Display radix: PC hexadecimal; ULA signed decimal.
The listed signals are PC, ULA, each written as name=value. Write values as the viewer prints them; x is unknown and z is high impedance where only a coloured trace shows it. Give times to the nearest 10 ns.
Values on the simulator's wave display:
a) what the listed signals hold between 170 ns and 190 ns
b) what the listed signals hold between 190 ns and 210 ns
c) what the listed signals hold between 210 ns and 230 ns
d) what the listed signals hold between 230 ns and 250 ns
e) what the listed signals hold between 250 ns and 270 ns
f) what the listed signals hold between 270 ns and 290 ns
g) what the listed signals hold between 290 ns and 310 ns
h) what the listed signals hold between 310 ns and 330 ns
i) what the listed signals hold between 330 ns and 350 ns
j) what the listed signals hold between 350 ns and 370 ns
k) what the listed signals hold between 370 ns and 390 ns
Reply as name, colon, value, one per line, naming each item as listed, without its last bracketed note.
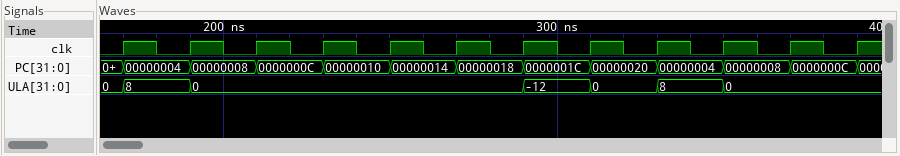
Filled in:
what the listed signals hold between 170 ns and 190 ns: PC=00000004, ULA=8
what the listed signals hold between 190 ns and 210 ns: PC=00000008, ULA=0
what the listed signals hold between 210 ns and 230 ns: PC=0000000C, ULA=0
what the listed signals hold between 230 ns and 250 ns: PC=00000010, ULA=0
what the listed signals hold between 250 ns and 270 ns: PC=00000014, ULA=0
what the listed signals hold between 270 ns and 290 ns: PC=00000018, ULA=0
what the listed signals hold between 290 ns and 310 ns: PC=0000001C, ULA=-12
what the listed signals hold between 310 ns and 330 ns: PC=00000020, ULA=0
what the listed signals hold between 330 ns and 350 ns: PC=00000004, ULA=8
what the listed signals hold between 350 ns and 370 ns: PC=00000008, ULA=0
what the listed signals hold between 370 ns and 390 ns: PC=0000000C, ULA=0
